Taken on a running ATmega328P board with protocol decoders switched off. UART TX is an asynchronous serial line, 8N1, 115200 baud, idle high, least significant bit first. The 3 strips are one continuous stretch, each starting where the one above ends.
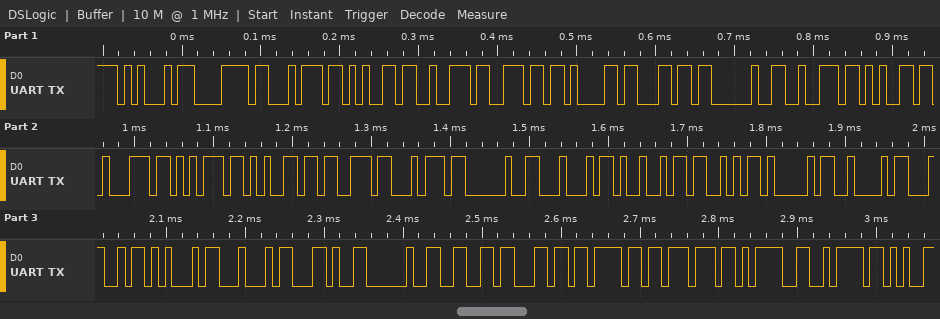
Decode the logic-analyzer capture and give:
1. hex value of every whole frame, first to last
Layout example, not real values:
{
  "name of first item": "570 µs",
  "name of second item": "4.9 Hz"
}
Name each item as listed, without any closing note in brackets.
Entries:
{
  "hex value of every whole frame, first to last": "45 78 74 65 72 6E 61 6C 20 72 65 71 75 65 73 74 20 44 49 53 41 42 4C 45 44 2C 20 66 6C 6F 77 3D 7A"
}
